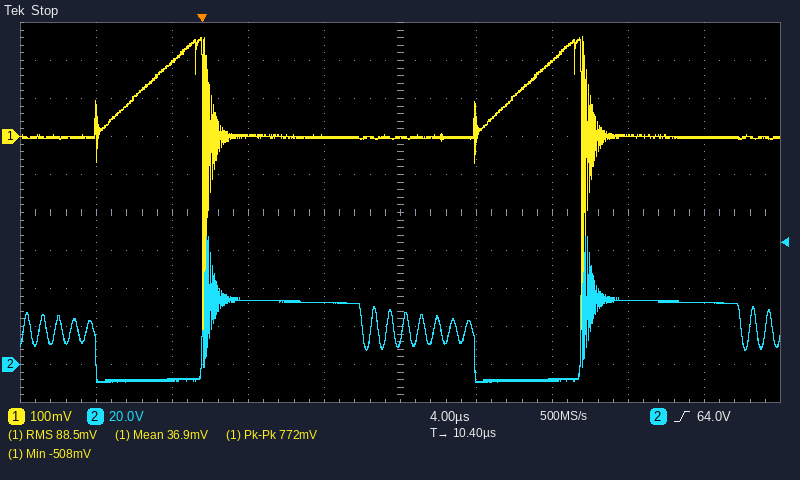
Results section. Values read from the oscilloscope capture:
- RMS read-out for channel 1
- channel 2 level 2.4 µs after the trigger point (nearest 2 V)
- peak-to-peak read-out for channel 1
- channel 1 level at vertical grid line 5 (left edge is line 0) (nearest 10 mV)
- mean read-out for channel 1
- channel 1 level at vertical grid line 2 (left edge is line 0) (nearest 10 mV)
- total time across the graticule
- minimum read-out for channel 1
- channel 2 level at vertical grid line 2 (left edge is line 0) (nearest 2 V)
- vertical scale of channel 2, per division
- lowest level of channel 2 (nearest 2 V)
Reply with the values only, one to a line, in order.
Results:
88.5 mV
34 V
772 mV
0 mV
36.9 mV
190 mV
40 µs
-508 mV
-8 V
20 V
-10 V
